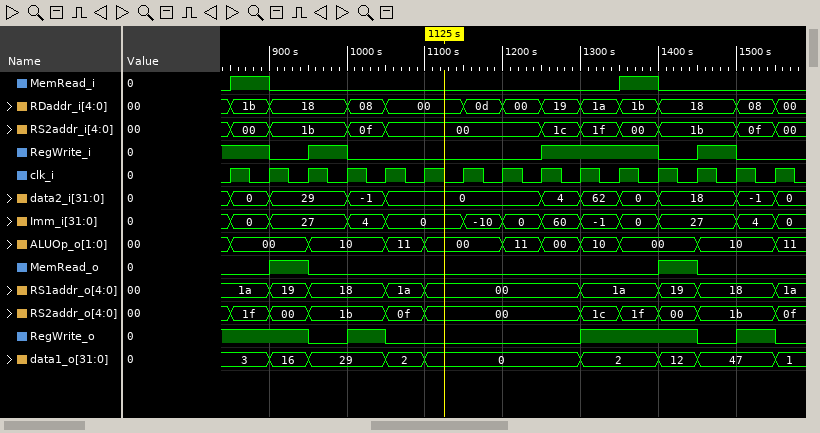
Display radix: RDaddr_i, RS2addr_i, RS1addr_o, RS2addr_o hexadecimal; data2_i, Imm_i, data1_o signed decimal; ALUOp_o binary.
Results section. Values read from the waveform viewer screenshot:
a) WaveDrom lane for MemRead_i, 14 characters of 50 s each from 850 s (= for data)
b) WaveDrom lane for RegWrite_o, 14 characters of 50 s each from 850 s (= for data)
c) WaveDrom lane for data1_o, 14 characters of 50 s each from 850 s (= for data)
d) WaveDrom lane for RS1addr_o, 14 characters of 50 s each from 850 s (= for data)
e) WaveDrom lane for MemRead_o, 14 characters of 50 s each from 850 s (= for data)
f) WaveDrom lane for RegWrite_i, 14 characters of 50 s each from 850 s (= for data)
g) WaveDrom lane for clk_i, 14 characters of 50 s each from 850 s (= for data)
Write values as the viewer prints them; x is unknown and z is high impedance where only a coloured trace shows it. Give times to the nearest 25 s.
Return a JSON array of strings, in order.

["{name: 'MemRead_i', wave: '10........10..'}", "{name: 'RegWrite_o', wave: '1.010....1..01'}", "{name: 'data1_o', wave: '===.==...=.==.', data: '3 16 29 2 0 2 12 47'}", "{name: 'RS1addr_o', wave: '===.==...=.==.', data: '1a 19 18 1a 00 1a 19 18'}", "{name: 'MemRead_o', wave: '010........10.'}", "{name: 'RegWrite_i', wave: '1010....1..010'}", "{name: 'clk_i', wave: 'p.............'}"]
